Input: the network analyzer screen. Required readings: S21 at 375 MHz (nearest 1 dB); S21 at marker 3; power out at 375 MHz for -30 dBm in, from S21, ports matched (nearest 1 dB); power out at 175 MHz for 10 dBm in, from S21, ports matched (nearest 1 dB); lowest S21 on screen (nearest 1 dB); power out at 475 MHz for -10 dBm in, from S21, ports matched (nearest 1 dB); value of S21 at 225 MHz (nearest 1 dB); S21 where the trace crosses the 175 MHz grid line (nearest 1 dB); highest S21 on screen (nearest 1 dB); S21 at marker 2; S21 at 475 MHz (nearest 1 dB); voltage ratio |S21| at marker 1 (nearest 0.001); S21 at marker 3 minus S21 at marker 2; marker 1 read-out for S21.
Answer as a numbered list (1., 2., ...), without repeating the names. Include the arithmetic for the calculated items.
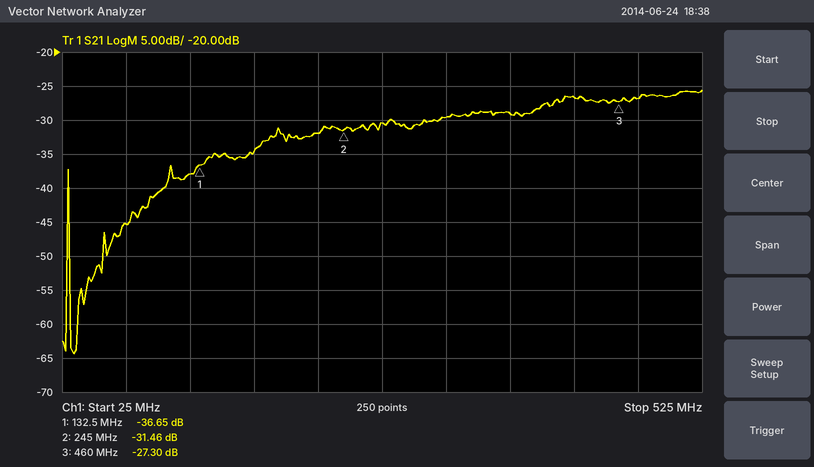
1. -29 dB
2. -27.30 dB
3. -30 dBm + (-29 dB) = -59 dBm
4. 10 dBm + (-35 dB) = -25 dBm
5. -64 dB
6. -10 dBm + (-27 dB) = -37 dBm
7. -32 dB
8. -35 dB
9. -26 dB
10. -31.46 dB
11. -27 dB
12. 10^(-36.65/20) ≈ 0.015
13. -27.3 − (-31.46) = 4.16 dB
14. -36.65 dB
